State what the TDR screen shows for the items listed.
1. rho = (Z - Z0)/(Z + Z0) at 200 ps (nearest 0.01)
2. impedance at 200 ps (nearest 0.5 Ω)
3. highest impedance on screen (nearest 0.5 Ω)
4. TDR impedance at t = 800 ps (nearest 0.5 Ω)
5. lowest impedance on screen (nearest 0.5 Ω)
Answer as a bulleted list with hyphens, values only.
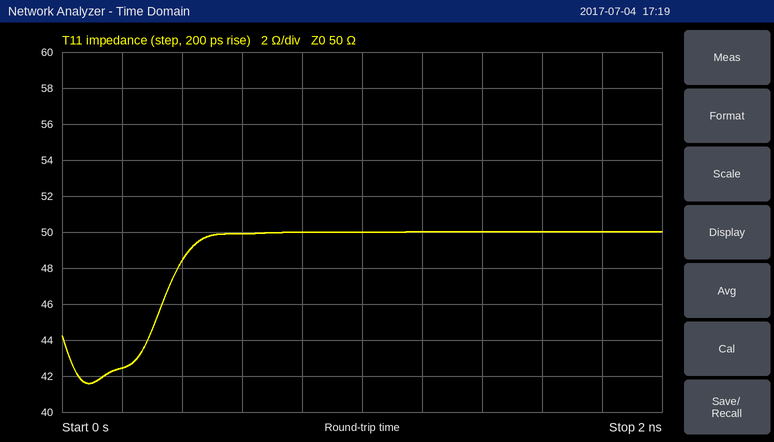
- -0.08
- 42.5 Ω
- 50.0 Ω
- 50.0 Ω
- 41.5 Ω
